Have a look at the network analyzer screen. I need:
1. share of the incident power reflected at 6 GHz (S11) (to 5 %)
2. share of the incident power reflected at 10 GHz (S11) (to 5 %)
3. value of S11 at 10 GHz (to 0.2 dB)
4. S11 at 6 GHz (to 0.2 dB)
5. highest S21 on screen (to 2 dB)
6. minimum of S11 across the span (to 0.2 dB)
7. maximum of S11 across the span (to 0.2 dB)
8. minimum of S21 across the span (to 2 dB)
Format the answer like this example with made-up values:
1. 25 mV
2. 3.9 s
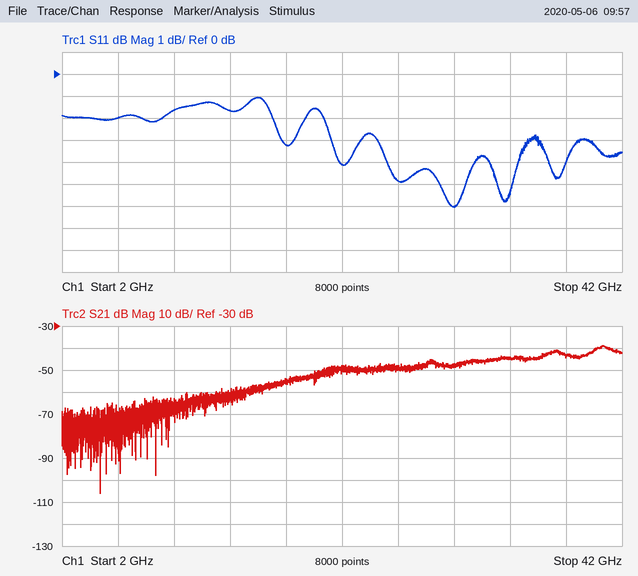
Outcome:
1. 65 %
2. 70 %
3. -1.6 dB
4. -2.0 dB
5. -38 dB
6. -6.0 dB
7. -1.0 dB
8. -106 dB
